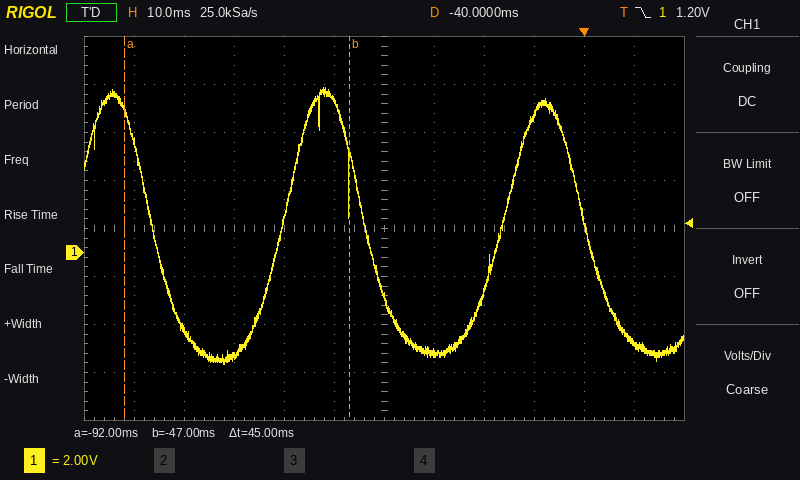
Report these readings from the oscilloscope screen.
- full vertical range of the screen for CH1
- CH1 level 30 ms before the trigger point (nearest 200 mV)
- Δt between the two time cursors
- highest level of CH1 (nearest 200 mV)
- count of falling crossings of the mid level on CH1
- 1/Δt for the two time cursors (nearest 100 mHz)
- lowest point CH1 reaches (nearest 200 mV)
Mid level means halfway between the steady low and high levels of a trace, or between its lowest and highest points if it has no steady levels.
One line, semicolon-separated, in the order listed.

16 V; -4.2 V; 45 ms; 6.8 V; 3; 22.2 Hz; -4.6 V
